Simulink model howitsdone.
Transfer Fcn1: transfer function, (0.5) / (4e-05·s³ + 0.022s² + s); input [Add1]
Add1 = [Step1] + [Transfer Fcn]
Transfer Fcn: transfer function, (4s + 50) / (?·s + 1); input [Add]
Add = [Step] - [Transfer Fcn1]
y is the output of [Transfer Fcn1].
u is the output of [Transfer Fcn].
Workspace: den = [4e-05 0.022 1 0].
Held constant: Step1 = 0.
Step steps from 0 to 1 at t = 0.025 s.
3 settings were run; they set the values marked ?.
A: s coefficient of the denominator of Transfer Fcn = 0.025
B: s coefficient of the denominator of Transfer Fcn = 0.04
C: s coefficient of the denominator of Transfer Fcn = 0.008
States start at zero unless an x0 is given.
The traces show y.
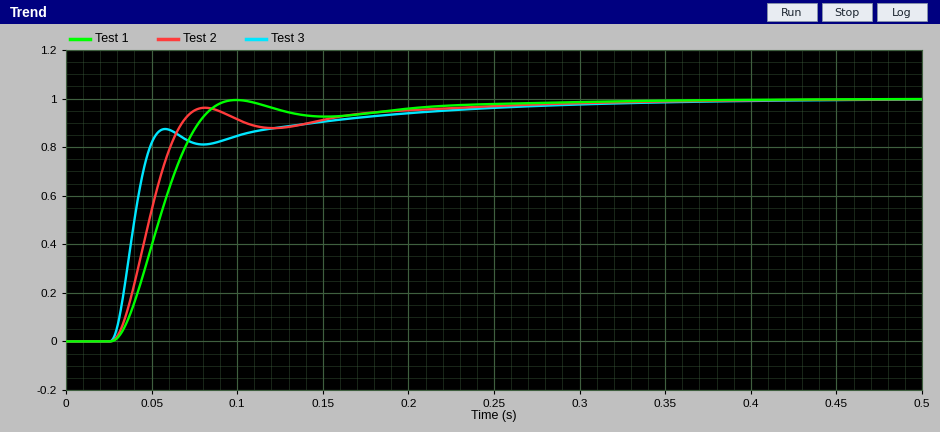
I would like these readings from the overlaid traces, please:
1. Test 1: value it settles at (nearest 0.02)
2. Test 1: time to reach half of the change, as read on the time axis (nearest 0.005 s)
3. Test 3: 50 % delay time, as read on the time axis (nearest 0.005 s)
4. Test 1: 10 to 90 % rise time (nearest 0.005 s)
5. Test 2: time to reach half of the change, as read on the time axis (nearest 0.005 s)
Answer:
1.00
0.055 s
0.040 s
0.040 s
0.050 s
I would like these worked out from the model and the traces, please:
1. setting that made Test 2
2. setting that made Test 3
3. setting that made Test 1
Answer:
A
C
B
